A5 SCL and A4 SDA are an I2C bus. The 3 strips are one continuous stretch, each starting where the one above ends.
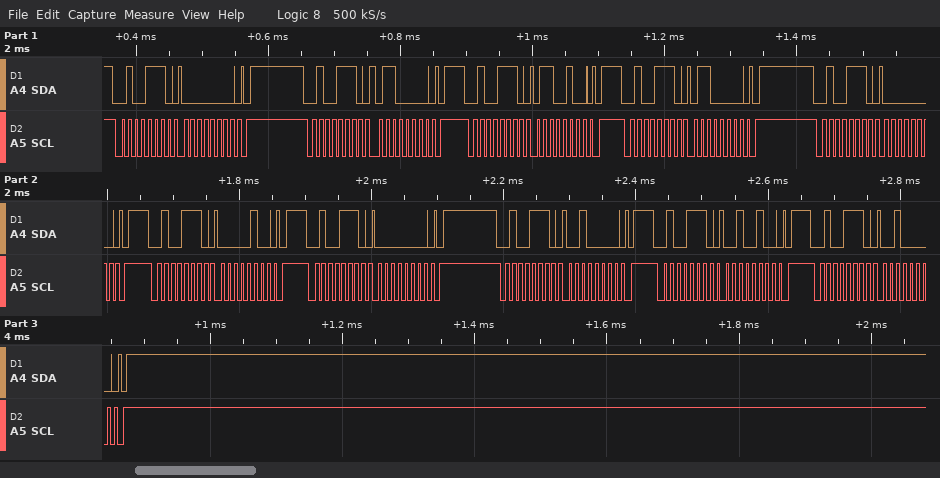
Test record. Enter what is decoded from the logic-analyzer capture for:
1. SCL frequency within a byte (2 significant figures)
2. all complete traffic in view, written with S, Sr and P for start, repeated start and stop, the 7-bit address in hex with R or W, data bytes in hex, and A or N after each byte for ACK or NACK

100 kHz
S 27W A 00 A P S 27W A 60 A P S 27W A 64 A P S 27W A 60 A P S 27W A 00 A P S 27W A 04 A P S 27W A 00 A P S 27W A 20 A P S 27W A 24 A P S 27W A 20 A P
